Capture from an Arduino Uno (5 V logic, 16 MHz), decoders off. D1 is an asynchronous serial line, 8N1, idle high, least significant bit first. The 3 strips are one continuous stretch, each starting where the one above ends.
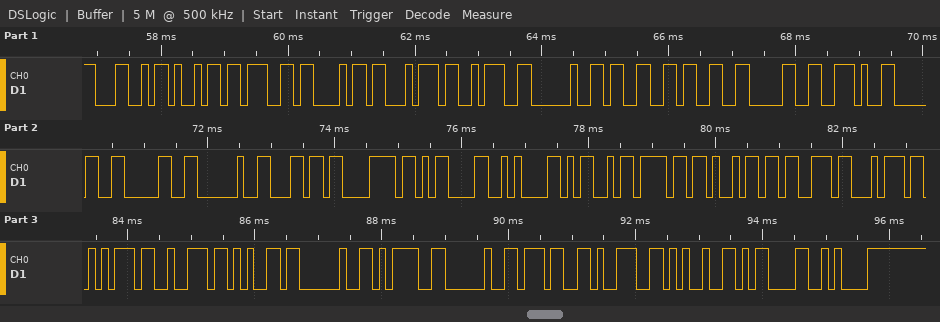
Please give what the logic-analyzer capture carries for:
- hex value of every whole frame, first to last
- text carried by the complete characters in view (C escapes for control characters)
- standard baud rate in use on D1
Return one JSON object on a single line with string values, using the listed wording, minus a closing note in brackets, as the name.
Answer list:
{"hex value of every whole frame, first to last": "4C 69 67 68 74 3A 20 33 33 30 2E 30 30 20 6C 78 0D 0A 4D 6F 69 73 74 75 72 65 20 3D 20 37 39 25 0D 0A", "text carried by the complete characters in view": "\"Light: 330.00 lx\\r\\nMoisture = 79%\\r\\n\"", "standard baud rate in use on D1": "9600 baud"}
